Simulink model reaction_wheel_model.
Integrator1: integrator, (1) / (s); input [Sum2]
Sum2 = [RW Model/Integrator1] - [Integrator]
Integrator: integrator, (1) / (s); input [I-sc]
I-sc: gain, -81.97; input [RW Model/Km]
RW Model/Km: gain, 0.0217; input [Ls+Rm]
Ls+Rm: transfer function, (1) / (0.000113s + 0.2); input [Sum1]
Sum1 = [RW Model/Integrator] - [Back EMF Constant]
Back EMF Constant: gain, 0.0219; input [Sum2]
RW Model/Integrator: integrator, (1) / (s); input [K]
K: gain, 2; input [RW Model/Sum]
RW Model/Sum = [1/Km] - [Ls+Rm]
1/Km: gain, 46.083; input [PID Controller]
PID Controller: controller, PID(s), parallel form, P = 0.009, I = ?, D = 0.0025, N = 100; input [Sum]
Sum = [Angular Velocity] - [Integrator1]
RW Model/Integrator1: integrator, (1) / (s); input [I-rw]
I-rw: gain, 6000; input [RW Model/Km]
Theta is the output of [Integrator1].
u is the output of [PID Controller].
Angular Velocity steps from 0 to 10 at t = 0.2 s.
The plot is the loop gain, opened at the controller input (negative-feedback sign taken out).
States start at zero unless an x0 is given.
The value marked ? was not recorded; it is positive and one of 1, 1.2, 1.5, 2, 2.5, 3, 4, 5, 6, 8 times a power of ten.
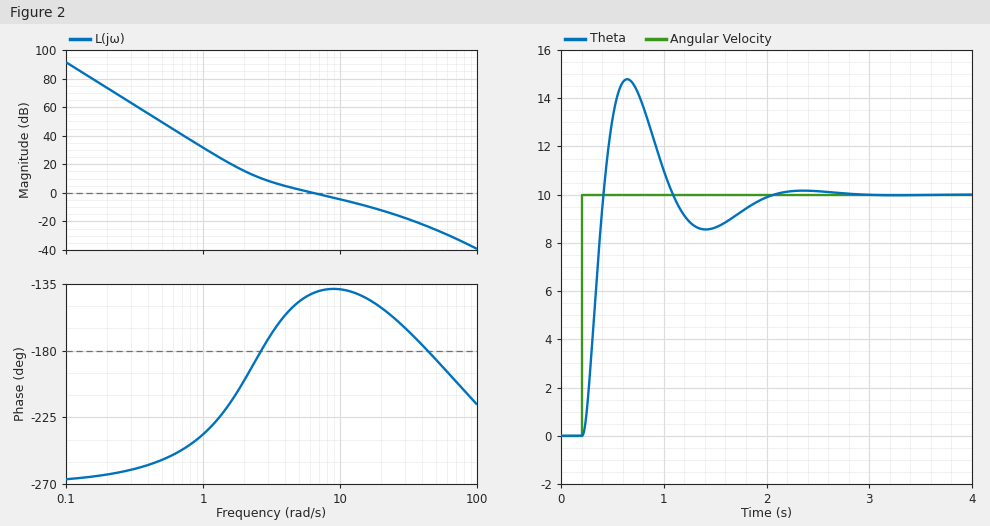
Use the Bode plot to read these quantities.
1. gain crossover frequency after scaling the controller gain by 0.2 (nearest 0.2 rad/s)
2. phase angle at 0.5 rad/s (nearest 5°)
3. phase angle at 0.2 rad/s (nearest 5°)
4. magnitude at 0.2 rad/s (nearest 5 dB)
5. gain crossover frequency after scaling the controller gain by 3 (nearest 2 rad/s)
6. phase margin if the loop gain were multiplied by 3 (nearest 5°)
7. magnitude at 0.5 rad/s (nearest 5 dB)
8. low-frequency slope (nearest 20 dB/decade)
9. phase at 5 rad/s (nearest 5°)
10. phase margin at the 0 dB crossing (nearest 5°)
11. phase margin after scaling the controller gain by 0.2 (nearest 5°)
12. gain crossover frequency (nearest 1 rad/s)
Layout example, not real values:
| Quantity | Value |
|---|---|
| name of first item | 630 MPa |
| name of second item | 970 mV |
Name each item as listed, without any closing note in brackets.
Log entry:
| Quantity | Value |
|---|---|
| gain crossover frequency after scaling the controller gain by 0.2 | 2.2 rad/s |
| phase angle at 0.5 rad/s | -255° |
| phase angle at 0.2 rad/s | -265° |
| magnitude at 0.2 rad/s | 75 dB |
| gain crossover frequency after scaling the controller gain by 3 | 16 rad/s |
| phase margin if the loop gain were multiplied by 3 | 35° |
| magnitude at 0.5 rad/s | 50 dB |
| low-frequency slope | -60 dB/decade |
| phase at 5 rad/s | -145° |
| phase margin at the 0 dB crossing | 40° |
| phase margin after scaling the controller gain by 0.2 | -15° |
| gain crossover frequency | 6 rad/s |
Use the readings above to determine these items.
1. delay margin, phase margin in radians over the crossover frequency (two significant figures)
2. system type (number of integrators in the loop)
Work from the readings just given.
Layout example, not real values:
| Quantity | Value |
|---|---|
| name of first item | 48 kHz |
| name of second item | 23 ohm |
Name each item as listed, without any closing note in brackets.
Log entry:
| Quantity | Value |
|---|---|
| delay margin, phase margin in radians over the crossover frequency | 0.12 s |
| system type | 3 |
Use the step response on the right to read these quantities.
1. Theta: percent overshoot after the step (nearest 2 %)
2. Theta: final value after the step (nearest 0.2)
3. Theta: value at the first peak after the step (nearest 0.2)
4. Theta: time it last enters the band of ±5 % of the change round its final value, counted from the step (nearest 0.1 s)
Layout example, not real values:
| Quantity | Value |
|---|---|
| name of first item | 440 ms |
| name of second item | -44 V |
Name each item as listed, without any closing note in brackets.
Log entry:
| Quantity | Value |
|---|---|
| Theta: percent overshoot after the step | 48 % |
| Theta: final value after the step | 10.0 |
| Theta: value at the first peak after the step | 14.8 |
| Theta: time it last enters the band of ±5 % of the change round its final value, counted from the step | 1.6 s |
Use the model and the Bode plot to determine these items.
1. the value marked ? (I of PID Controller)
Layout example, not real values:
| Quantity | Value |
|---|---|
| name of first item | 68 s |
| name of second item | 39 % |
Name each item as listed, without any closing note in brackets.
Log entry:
| Quantity | Value |
|---|---|
| the value marked ? | 0.015 |
